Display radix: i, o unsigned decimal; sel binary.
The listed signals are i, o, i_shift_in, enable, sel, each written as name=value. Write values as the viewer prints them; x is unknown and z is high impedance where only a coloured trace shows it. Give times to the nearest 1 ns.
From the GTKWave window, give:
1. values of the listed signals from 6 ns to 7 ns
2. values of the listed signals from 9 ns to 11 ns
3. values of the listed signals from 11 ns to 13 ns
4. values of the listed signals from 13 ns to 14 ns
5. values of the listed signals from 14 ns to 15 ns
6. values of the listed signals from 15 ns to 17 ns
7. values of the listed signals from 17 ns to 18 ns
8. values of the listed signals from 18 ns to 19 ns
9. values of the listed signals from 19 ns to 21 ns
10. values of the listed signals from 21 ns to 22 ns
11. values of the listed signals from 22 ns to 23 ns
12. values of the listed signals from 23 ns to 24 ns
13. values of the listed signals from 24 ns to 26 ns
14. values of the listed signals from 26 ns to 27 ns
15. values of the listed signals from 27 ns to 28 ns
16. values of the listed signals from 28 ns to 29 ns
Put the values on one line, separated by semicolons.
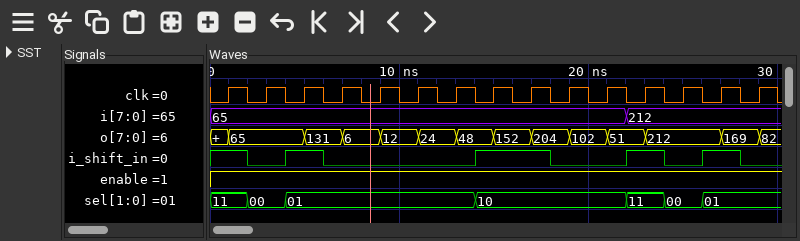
i=65, o=131, i_shift_in=0, enable=1, sel=01; i=65, o=12, i_shift_in=0, enable=1, sel=01; i=65, o=24, i_shift_in=0, enable=1, sel=01; i=65, o=48, i_shift_in=0, enable=1, sel=01; i=65, o=48, i_shift_in=1, enable=1, sel=10; i=65, o=152, i_shift_in=1, enable=1, sel=10; i=65, o=204, i_shift_in=1, enable=1, sel=10; i=65, o=204, i_shift_in=0, enable=1, sel=10; i=65, o=102, i_shift_in=0, enable=1, sel=10; i=65, o=51, i_shift_in=0, enable=1, sel=10; i=212, o=51, i_shift_in=1, enable=1, sel=11; i=212, o=212, i_shift_in=1, enable=1, sel=11; i=212, o=212, i_shift_in=0, enable=1, sel=00; i=212, o=212, i_shift_in=1, enable=1, sel=01; i=212, o=169, i_shift_in=1, enable=1, sel=01; i=212, o=169, i_shift_in=0, enable=1, sel=01
